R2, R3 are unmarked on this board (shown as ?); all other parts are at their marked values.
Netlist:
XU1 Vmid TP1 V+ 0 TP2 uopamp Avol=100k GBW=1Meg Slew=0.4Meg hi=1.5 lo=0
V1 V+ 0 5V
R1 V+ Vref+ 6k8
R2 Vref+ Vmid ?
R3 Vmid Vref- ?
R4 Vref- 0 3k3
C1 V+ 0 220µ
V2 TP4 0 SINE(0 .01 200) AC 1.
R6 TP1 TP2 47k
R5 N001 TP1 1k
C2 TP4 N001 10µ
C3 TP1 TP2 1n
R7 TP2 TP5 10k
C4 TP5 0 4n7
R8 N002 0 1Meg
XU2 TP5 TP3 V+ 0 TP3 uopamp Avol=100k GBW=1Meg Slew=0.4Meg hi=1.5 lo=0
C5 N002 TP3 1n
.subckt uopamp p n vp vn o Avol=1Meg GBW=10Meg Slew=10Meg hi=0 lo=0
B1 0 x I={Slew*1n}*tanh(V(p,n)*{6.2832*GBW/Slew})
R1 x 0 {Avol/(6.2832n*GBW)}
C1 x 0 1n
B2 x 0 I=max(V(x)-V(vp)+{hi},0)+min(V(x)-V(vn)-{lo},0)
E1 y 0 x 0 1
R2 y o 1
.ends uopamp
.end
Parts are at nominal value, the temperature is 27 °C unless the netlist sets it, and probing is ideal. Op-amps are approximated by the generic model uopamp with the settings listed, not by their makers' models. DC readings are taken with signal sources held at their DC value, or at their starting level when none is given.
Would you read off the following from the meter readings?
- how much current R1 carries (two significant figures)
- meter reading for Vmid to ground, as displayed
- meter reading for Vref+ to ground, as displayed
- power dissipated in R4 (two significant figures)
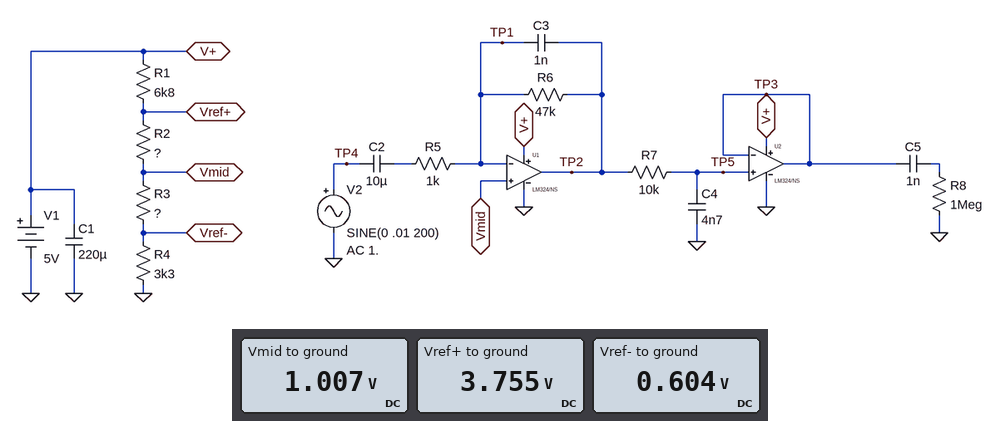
180 µA
1.007 V
3.755 V
110 µW
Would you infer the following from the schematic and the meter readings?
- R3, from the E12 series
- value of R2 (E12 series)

2.2 kΩ
15 kΩ
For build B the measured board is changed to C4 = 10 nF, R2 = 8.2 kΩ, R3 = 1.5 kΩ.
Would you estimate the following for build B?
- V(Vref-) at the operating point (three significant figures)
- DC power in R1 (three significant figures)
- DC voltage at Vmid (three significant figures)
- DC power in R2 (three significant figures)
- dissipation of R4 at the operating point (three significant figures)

833 mV
434 µW
1.21 V
523 µW
210 µW
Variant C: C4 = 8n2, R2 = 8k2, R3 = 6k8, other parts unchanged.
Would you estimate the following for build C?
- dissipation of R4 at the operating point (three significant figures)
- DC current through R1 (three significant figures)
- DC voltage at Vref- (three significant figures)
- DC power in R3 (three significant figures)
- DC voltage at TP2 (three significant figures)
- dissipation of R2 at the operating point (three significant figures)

131 µW
199 µA
657 mV
270 µW
2.01 V
325 µW
